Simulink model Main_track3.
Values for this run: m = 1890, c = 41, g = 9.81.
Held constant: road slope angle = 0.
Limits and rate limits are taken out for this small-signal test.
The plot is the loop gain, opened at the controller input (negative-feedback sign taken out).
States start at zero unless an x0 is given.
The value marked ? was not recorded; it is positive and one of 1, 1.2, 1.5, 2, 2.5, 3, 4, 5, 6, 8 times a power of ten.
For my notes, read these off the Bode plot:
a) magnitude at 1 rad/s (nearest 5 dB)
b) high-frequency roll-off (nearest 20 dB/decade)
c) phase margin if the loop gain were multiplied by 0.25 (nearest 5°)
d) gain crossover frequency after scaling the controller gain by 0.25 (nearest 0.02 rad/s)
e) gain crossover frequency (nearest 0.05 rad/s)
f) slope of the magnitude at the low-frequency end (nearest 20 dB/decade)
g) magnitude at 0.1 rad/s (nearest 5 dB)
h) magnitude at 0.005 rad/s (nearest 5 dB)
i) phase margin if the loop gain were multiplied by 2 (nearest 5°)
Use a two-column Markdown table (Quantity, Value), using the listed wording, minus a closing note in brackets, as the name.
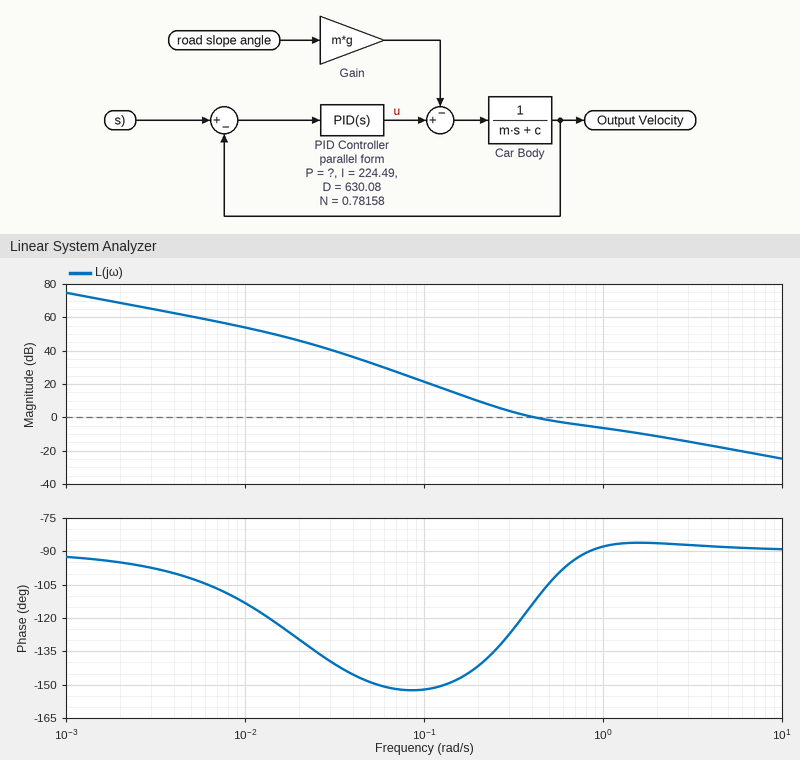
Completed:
| Quantity | Value |
|---|---|
| magnitude at 1 rad/s | -5 dB |
| high-frequency roll-off | -20 dB/decade |
| phase margin if the loop gain were multiplied by 0.25 | 35° |
| gain crossover frequency after scaling the controller gain by 0.25 | 0.18 rad/s |
| gain crossover frequency | 0.40 rad/s |
| slope of the magnitude at the low-frequency end | -20 dB/decade |
| magnitude at 0.1 rad/s | 20 dB |
| magnitude at 0.005 rad/s | 60 dB |
| phase margin if the loop gain were multiplied by 2 | 90° |
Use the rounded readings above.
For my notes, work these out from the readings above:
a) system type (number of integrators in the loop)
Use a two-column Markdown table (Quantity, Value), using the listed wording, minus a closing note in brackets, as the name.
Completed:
| Quantity | Value |
|---|---|
| system type | 1 |
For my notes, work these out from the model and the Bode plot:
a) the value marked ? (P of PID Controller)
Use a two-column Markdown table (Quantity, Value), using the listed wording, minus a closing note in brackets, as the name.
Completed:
| Quantity | Value |
|---|---|
| the value marked ? | 600 |
